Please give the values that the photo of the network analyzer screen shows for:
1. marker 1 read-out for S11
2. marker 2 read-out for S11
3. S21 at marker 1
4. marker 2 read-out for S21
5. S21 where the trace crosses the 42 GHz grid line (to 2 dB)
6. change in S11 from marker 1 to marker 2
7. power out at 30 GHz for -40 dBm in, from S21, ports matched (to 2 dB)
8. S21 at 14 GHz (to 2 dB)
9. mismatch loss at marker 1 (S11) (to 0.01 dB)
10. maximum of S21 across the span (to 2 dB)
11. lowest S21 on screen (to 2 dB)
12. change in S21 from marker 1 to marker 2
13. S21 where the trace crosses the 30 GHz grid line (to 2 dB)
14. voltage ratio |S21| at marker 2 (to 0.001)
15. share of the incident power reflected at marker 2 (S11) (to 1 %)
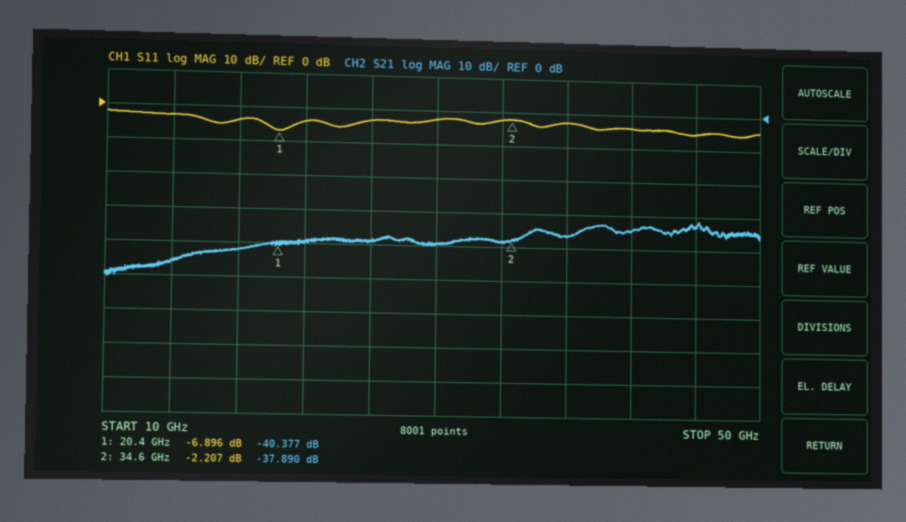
-6.896 dB
-2.207 dB
-40.377 dB
-37.890 dB
-34 dB
4.689 dB
-80 dBm
-46 dB
0.99 dB
-32 dB
-50 dB
2.487 dB
-40 dB
0.013
60 %
